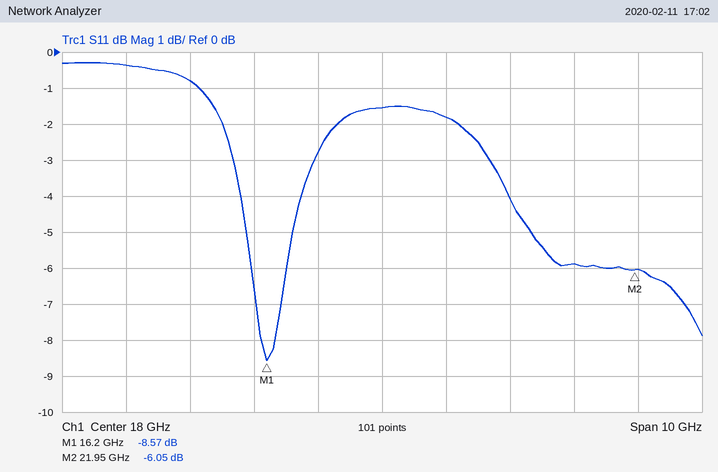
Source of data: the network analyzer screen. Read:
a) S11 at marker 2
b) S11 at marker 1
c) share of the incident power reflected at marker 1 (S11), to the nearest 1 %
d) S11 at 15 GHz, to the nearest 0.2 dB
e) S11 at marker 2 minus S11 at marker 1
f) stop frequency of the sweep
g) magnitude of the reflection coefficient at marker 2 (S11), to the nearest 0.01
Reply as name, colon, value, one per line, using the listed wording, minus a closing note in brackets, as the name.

S11 at marker 2: -6.05 dB
S11 at marker 1: -8.57 dB
share of the incident power reflected at marker 1 (S11), to the nearest 1 %: 14 %
S11 at 15 GHz, to the nearest 0.2 dB: -0.8 dB
S11 at marker 2 minus S11 at marker 1: 2.52 dB
stop frequency of the sweep: 23 GHz
magnitude of the reflection coefficient at marker 2 (S11), to the nearest 0.01: 0.50
